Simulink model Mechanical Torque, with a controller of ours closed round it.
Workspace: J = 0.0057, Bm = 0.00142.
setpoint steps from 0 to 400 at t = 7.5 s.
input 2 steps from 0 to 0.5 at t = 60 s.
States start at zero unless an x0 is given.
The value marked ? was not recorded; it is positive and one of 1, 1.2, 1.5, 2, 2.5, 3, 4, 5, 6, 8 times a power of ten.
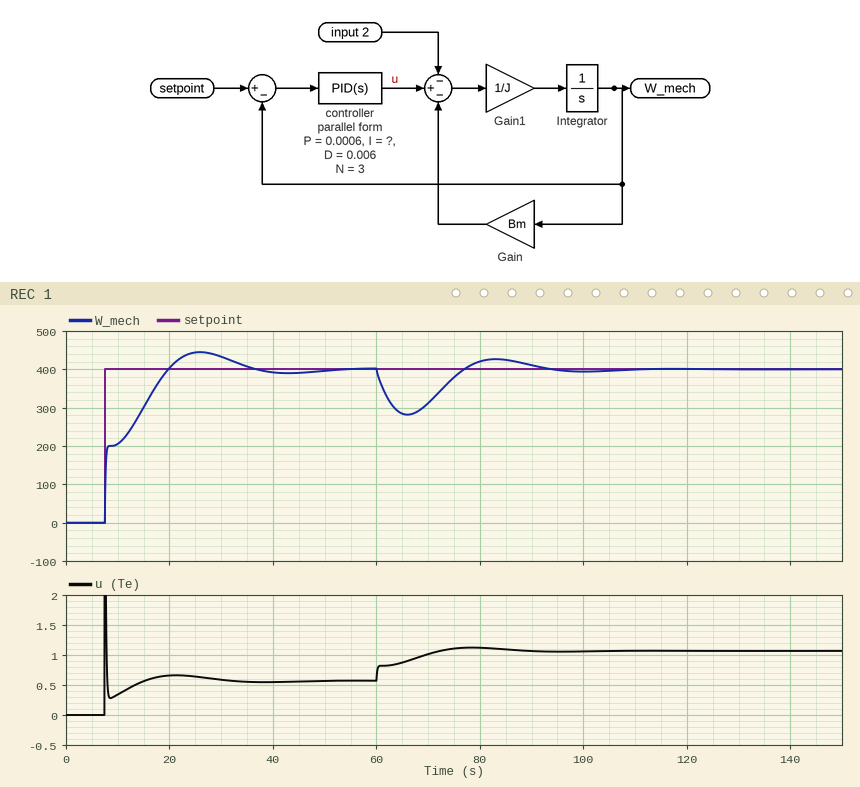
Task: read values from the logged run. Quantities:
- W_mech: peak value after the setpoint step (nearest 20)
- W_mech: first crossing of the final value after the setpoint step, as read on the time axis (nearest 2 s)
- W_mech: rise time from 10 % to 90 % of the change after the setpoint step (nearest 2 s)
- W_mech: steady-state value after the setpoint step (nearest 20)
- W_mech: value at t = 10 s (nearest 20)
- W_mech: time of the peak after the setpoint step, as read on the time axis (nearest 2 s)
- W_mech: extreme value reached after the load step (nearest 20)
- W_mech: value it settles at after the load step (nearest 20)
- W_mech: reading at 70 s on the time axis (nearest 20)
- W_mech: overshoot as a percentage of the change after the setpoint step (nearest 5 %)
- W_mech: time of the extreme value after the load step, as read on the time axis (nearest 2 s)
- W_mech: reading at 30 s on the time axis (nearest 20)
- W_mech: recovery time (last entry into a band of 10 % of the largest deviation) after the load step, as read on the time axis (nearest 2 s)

440
20 s
10 s
400
200
26 s
280
400
320
10 %
66 s
440
90 s
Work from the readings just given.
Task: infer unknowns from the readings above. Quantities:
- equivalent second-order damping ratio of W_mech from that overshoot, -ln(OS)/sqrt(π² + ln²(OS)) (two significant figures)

0.59
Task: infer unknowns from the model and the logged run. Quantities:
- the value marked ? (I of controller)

0.0005
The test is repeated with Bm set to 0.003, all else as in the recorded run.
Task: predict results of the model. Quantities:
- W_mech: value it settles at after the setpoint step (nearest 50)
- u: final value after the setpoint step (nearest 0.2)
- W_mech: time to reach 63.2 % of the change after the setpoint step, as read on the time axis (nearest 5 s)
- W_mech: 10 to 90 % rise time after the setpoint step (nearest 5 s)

400
1.2
15 s
15 s
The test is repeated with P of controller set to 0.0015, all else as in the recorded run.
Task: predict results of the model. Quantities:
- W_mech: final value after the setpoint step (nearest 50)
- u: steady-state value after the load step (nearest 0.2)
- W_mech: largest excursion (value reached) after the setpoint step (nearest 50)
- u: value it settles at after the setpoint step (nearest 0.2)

400
1.0
400
0.6
